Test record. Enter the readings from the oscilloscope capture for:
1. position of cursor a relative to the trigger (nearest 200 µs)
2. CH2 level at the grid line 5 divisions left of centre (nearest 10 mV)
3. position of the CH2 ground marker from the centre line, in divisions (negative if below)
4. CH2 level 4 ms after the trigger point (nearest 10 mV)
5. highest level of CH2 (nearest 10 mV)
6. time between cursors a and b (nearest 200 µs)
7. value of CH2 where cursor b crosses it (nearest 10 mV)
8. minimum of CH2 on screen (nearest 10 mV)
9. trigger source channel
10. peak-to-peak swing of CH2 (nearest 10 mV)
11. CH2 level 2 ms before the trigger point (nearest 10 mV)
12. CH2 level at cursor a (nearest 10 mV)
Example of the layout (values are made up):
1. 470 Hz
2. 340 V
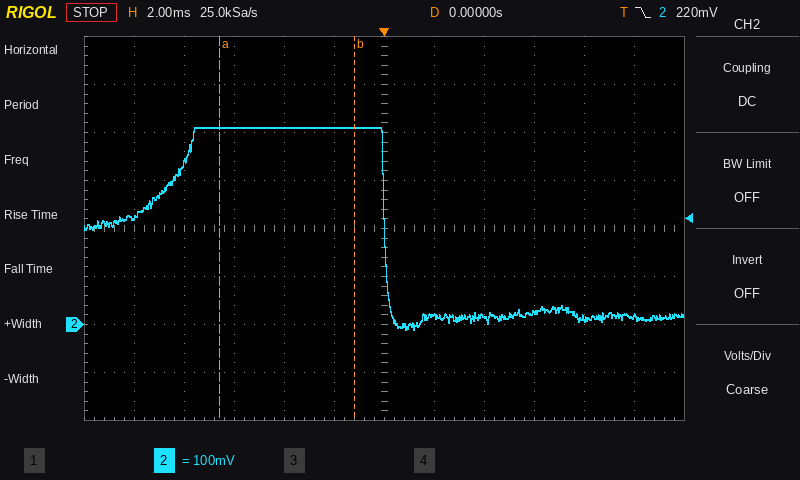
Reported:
1. -6.6 ms
2. 220 mV
3. -2.0 div
4. 20 mV
5. 410 mV
6. 5.4 ms
7. 410 mV
8. -10 mV
9. CH2
10. 420 mV
11. 410 mV
12. 410 mV
